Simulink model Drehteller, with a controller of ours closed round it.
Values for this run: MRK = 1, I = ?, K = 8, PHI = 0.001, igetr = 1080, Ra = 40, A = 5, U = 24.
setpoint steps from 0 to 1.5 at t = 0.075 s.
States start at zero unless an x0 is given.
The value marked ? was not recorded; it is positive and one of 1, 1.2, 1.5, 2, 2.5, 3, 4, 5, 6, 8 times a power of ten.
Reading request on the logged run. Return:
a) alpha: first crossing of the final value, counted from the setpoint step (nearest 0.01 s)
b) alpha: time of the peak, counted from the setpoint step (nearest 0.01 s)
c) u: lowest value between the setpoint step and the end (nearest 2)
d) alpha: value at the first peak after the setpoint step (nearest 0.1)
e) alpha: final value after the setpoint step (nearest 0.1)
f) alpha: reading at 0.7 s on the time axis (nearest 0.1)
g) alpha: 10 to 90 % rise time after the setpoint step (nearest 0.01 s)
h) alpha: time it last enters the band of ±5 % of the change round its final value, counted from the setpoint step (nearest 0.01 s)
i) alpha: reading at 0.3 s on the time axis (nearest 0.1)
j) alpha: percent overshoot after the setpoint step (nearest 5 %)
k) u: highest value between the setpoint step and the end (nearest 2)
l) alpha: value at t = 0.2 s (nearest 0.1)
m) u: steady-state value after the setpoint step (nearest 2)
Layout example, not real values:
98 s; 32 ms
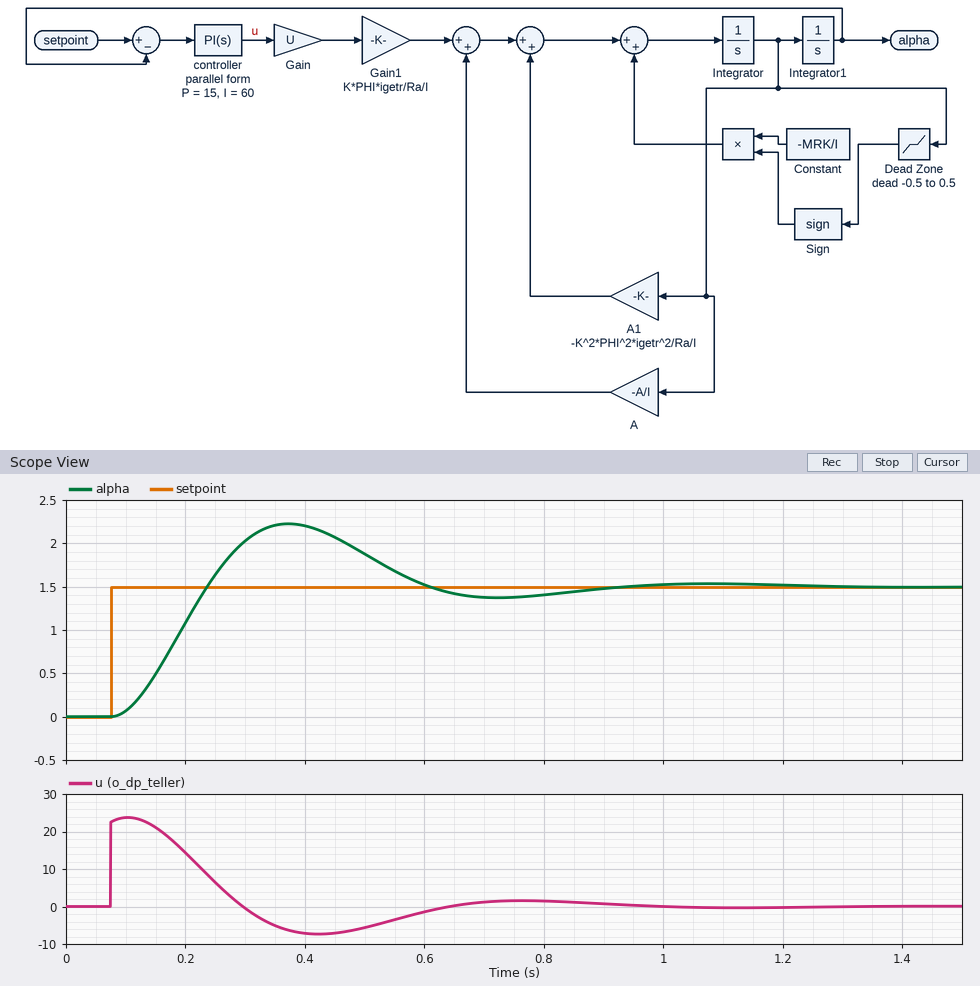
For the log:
0.16 s; 0.30 s; -8; 2.2; 1.5; 1.4; 0.11 s; 0.75 s; 2.0; 50 %; 24; 1.1; 0
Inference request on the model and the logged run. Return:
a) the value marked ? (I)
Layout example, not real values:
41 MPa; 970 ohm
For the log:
0.5
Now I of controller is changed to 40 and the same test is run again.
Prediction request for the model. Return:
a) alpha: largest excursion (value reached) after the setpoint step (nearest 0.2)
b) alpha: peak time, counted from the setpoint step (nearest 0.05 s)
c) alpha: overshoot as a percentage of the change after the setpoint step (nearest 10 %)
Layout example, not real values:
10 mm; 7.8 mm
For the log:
2.0; 0.30 s; 40 %
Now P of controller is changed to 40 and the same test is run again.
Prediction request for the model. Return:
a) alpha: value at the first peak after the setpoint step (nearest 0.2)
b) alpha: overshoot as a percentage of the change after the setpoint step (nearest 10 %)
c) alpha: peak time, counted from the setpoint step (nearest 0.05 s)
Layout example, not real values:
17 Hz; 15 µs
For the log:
2.2; 40 %; 0.15 s
